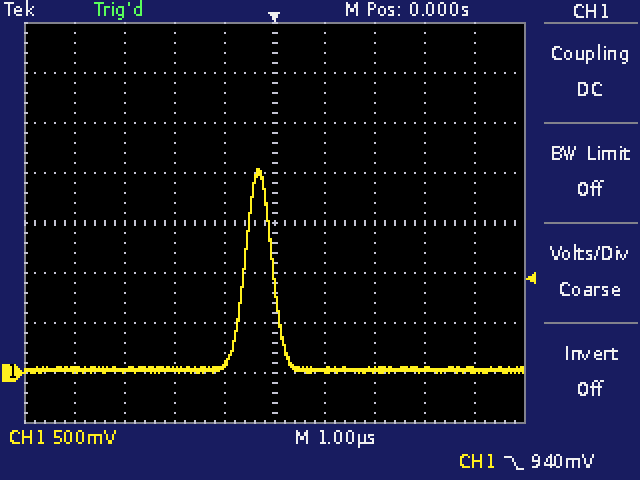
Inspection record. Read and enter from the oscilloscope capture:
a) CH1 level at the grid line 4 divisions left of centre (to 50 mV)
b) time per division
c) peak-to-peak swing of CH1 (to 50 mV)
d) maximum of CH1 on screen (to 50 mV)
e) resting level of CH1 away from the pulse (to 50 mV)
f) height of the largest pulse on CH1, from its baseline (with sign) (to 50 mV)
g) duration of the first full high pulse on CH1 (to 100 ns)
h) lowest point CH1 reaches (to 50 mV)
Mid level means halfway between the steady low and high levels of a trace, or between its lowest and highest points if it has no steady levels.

50 mV
1 µs
2.05 V
2.05 V
50 mV
+2.00 V
600 ns
0 mV
